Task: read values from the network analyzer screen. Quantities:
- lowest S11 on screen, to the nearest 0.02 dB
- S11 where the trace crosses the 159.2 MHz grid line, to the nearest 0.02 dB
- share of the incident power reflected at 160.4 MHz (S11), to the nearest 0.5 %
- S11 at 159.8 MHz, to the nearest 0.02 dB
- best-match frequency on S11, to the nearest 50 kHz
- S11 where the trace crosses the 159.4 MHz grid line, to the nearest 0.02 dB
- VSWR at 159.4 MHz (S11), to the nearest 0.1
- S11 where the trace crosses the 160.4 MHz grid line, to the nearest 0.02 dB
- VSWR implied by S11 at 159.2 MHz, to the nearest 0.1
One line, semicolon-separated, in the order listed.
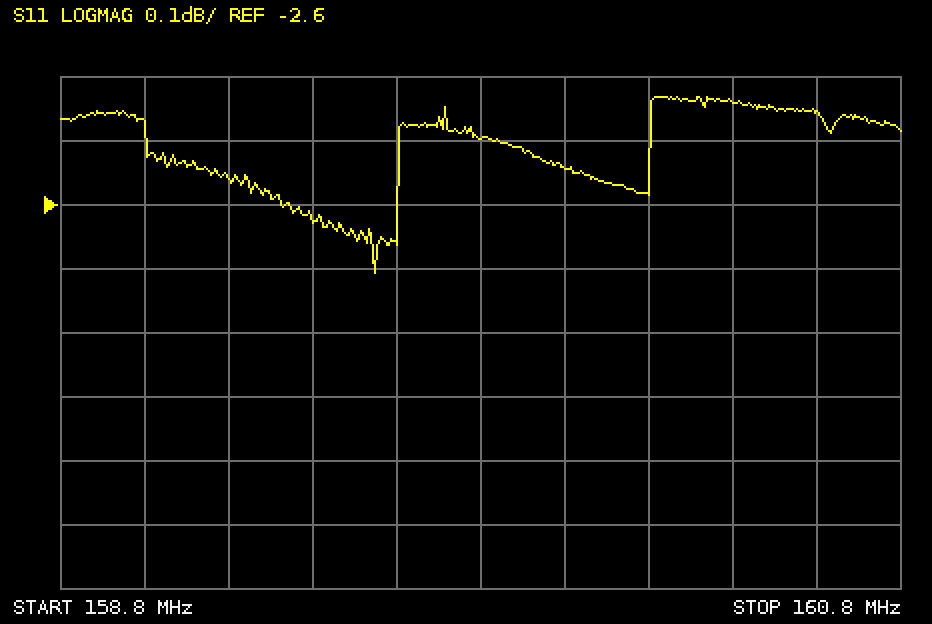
-2.70 dB; -2.56 dB; 57.0 %; -2.50 dB; 159.55 MHz; -2.62 dB; 6.7; -2.44 dB; 6.8
